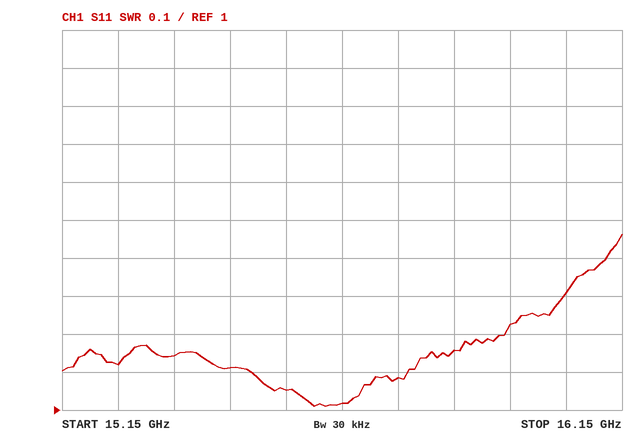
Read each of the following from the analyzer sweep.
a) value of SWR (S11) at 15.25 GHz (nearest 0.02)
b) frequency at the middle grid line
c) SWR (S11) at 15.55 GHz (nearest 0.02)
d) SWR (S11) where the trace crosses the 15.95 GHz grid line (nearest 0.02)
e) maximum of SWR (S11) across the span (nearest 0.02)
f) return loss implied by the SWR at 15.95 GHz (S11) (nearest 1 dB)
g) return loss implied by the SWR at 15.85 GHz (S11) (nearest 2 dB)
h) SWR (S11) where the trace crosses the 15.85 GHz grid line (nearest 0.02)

1.12
15.65 GHz
1.06
1.22
1.46
20 dB
22 dB
1.16
